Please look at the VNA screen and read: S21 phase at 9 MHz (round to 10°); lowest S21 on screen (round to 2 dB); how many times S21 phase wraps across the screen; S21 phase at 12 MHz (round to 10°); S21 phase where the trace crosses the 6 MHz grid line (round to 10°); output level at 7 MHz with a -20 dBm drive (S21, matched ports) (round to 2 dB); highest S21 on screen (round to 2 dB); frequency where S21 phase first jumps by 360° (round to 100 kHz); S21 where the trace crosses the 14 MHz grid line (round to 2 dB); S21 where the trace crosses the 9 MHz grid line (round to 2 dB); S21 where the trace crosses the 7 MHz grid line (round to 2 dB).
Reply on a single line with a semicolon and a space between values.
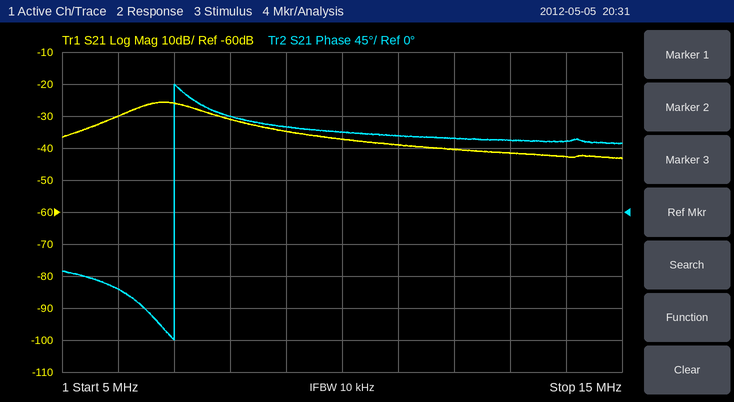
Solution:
120°; -44 dB; 1; 100°; -110°; -46 dBm; -26 dB; 7.0 MHz; -42 dB; -34 dB; -26 dB
